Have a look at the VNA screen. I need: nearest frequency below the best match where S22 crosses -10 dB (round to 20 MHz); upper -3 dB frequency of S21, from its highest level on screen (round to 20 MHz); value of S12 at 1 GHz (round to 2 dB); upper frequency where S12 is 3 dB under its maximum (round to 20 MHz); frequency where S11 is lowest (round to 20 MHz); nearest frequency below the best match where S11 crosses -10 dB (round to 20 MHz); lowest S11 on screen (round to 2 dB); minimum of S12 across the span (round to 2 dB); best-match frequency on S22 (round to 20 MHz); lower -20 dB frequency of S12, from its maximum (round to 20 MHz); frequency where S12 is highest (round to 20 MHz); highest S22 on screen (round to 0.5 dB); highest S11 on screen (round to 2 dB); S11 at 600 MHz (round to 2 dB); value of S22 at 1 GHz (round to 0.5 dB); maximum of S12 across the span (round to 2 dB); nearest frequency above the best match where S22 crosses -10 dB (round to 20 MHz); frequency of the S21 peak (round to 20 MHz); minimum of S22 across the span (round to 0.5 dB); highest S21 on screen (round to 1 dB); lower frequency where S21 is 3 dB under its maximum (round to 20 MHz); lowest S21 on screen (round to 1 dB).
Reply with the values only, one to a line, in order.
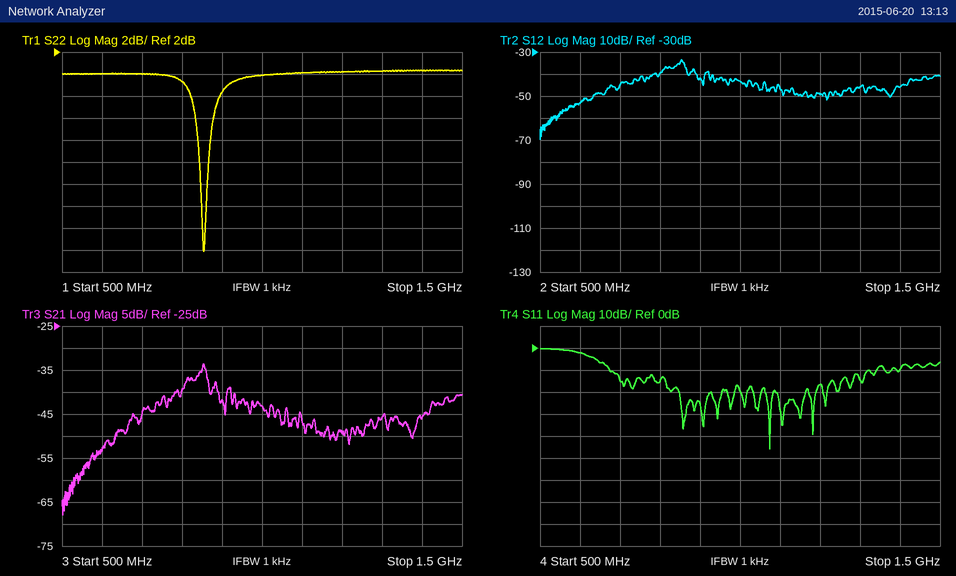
840 MHz
860 MHz
-44 dB
860 MHz
1.08 GHz
680 MHz
-46 dB
-70 dB
860 MHz
600 MHz
860 MHz
0.5 dB
0 dB
-2 dB
0.0 dB
-34 dB
860 MHz
860 MHz
-16.0 dB
-34 dB
840 MHz
-68 dB
